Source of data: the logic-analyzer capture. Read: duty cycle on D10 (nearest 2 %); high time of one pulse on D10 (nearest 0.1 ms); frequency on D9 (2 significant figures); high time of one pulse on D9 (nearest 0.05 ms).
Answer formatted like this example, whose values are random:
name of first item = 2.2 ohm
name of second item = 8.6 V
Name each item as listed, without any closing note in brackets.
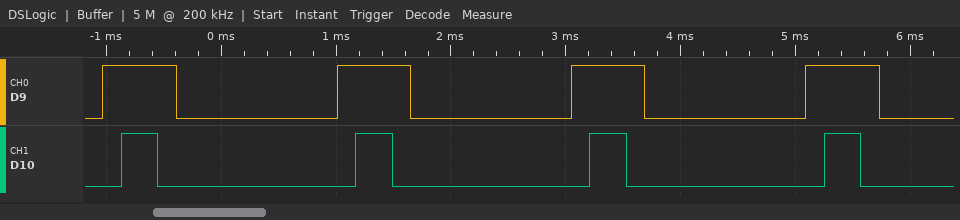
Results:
duty cycle on D10 = 16 %
high time of one pulse on D10 = 0.3 ms
frequency on D9 = 490 Hz
high time of one pulse on D9 = 0.65 ms
